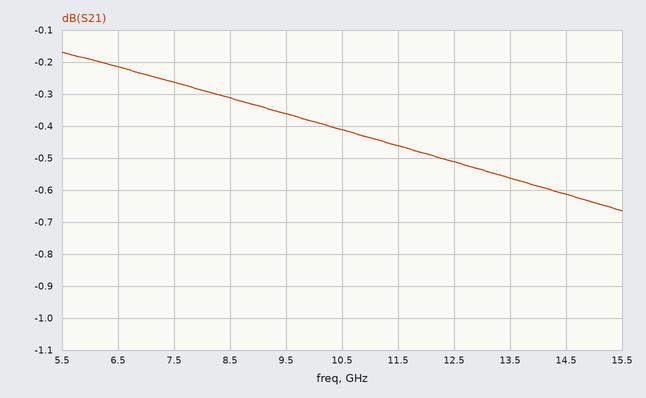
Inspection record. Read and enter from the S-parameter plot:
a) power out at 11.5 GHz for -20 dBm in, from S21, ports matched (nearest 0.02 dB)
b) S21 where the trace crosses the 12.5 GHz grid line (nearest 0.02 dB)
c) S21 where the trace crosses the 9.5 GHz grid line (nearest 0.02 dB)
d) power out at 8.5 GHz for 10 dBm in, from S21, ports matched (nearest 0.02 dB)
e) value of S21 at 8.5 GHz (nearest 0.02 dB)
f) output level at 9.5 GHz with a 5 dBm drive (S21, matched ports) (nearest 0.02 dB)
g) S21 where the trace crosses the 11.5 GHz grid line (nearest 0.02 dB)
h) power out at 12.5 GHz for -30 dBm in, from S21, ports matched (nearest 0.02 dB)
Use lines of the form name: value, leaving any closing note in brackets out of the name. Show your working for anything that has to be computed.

power out at 11.5 GHz for -20 dBm in, from S21, ports matched: -20 dBm + (-0.46 dB) = -20.46 dBm
S21 where the trace crosses the 12.5 GHz grid line: -0.52 dB
S21 where the trace crosses the 9.5 GHz grid line: -0.36 dB
power out at 8.5 GHz for 10 dBm in, from S21, ports matched: 10 dBm + (-0.32 dB) = 9.68 dBm
value of S21 at 8.5 GHz: -0.32 dB
output level at 9.5 GHz with a 5 dBm drive (S21, matched ports): 5 dBm + (-0.36 dB) = 4.64 dBm
S21 where the trace crosses the 11.5 GHz grid line: -0.46 dB
power out at 12.5 GHz for -30 dBm in, from S21, ports matched: -30 dBm + (-0.52 dB) = -30.52 dBm
